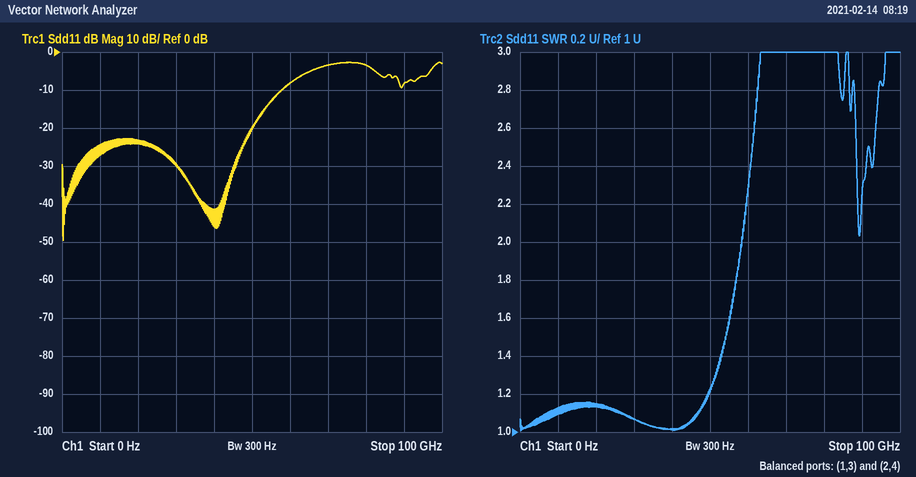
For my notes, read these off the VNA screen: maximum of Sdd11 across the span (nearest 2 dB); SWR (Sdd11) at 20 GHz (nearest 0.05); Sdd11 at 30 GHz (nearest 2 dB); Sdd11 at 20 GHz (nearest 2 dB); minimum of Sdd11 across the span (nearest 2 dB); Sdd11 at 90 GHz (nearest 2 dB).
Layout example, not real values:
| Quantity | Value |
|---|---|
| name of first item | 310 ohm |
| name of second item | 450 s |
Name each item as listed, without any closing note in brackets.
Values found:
| Quantity | Value |
|---|---|
| maximum of Sdd11 across the span | -2 dB |
| SWR (Sdd11) at 20 GHz | 1.15 |
| Sdd11 at 30 GHz | -30 dB |
| Sdd11 at 20 GHz | -24 dB |
| minimum of Sdd11 across the span | -50 dB |
| Sdd11 at 90 GHz | -8 dB |
